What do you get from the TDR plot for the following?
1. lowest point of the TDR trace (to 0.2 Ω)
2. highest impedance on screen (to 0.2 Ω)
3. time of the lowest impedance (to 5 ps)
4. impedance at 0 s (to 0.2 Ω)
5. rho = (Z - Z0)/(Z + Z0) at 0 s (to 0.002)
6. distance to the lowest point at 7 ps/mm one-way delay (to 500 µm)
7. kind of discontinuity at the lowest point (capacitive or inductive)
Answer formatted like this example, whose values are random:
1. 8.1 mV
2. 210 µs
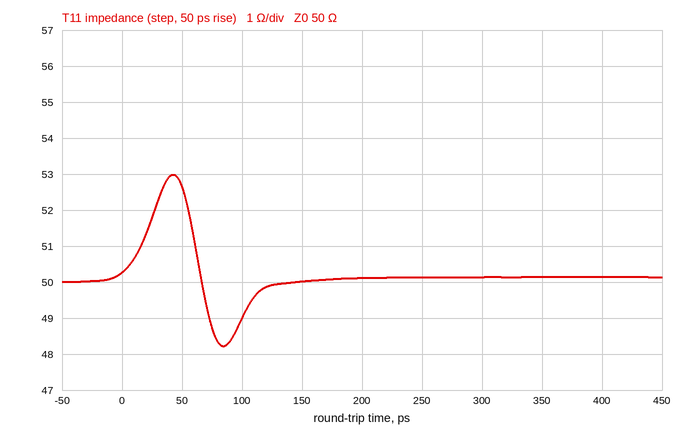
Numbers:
1. 48.2 Ω
2. 53.0 Ω
3. 85 ps
4. 50.2 Ω
5. +0.002
6. 6.0 mm
7. capacitive
